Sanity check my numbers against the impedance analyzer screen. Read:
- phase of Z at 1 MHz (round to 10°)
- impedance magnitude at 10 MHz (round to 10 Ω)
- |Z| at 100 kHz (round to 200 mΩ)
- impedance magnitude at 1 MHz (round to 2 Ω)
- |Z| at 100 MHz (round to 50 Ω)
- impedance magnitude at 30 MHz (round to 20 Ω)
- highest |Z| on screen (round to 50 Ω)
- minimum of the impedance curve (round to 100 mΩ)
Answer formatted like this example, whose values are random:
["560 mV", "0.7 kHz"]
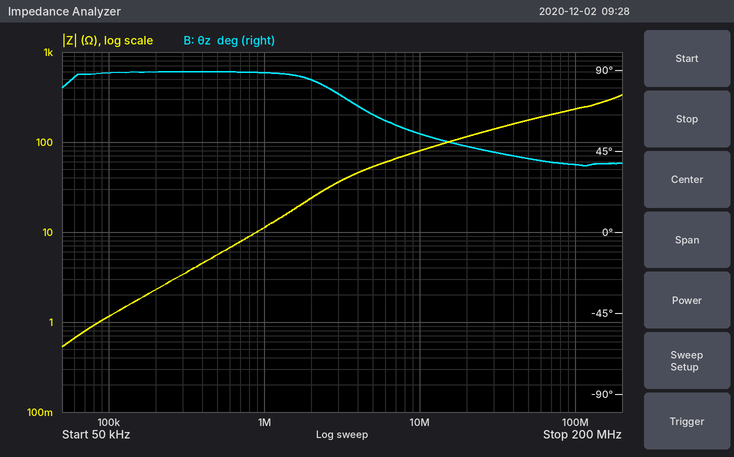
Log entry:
["90°", "80 Ω", "1.2 Ω", "12 Ω", "250 Ω", "140 Ω", "350 Ω", "500 mΩ"]
